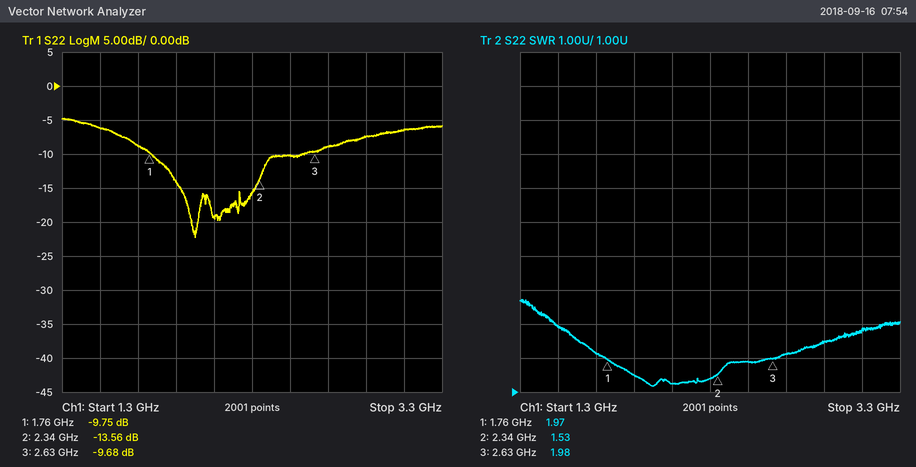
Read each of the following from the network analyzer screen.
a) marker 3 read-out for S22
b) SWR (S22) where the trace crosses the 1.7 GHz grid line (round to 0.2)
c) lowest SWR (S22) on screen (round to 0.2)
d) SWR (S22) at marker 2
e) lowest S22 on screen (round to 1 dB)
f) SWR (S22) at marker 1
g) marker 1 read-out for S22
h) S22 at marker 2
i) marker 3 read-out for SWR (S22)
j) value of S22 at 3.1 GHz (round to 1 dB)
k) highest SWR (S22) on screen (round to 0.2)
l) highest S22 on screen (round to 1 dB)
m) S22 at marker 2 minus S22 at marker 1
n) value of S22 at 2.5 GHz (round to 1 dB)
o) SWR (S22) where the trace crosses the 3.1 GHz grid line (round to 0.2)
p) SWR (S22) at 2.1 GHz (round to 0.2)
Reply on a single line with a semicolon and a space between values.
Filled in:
-9.68 dB; 2.2; 1.2; 1.53; -22 dB; 1.97; -9.75 dB; -13.56 dB; 1.98; -6 dB; 3.8; -5 dB; -3.81 dB; -10 dB; 2.8; 1.2
